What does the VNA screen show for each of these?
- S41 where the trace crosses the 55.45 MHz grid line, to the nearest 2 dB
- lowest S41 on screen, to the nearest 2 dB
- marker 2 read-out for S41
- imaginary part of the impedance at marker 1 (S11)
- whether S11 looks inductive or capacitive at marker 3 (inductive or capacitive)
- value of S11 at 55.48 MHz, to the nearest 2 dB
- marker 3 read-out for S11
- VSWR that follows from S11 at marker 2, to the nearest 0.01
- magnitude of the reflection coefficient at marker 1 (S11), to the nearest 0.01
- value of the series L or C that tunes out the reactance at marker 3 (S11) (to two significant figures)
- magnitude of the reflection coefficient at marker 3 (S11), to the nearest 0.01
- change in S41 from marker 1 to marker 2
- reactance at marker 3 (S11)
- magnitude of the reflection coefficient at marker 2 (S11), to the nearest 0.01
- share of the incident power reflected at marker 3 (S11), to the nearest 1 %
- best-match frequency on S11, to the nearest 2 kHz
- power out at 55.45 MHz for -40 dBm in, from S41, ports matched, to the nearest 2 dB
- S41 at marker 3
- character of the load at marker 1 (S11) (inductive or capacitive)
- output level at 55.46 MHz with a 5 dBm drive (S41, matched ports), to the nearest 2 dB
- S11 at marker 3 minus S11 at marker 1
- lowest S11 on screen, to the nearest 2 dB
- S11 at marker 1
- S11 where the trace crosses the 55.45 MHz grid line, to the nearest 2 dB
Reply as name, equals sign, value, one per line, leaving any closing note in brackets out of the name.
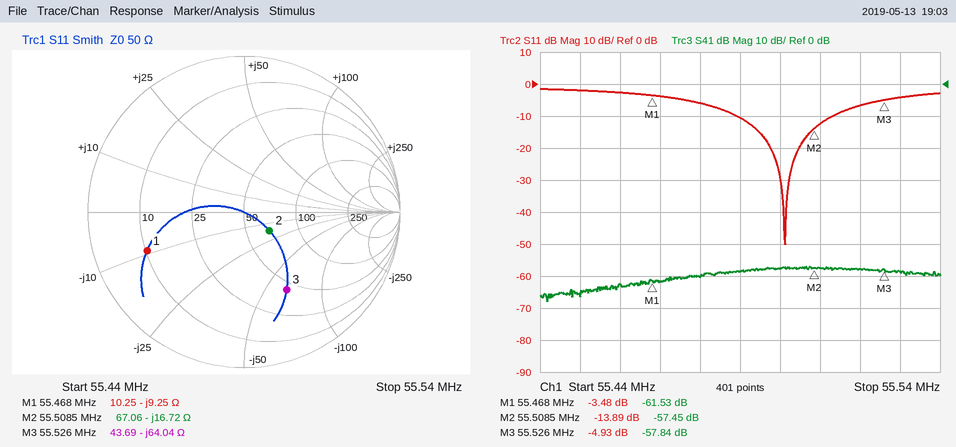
S41 where the trace crosses the 55.45 MHz grid line, to the nearest 2 dB = -66 dB
lowest S41 on screen, to the nearest 2 dB = -68 dB
marker 2 read-out for S41 = -57.45 dB
imaginary part of the impedance at marker 1 = -9.25 Ω
whether S11 looks inductive or capacitive at marker 3 = capacitive
value of S11 at 55.48 MHz, to the nearest 2 dB = -6 dB
marker 3 read-out for S11 = -4.93 dB
VSWR that follows from S11 at marker 2, to the nearest 0.01 = 1.51
magnitude of the reflection coefficient at marker 1 (S11), to the nearest 0.01 = 0.67
value of the series L or C that tunes out the reactance at marker 3 (S11) = 180 nH
magnitude of the reflection coefficient at marker 3 (S11), to the nearest 0.01 = 0.57
change in S41 from marker 1 to marker 2 = 4.08 dB
reactance at marker 3 = -64.04 Ω
magnitude of the reflection coefficient at marker 2 (S11), to the nearest 0.01 = 0.20
share of the incident power reflected at marker 3 (S11), to the nearest 1 % = 32 %
best-match frequency on S11, to the nearest 2 kHz = 55.502 MHz
power out at 55.45 MHz for -40 dBm in, from S41, ports matched, to the nearest 2 dB = -106 dBm
S41 at marker 3 = -57.84 dB
character of the load at marker 1 (S11) = capacitive
output level at 55.46 MHz with a 5 dBm drive (S41, matched ports), to the nearest 2 dB = -58 dBm
S11 at marker 3 minus S11 at marker 1 = -1.45 dB
lowest S11 on screen, to the nearest 2 dB = -50 dB
S11 at marker 1 = -3.48 dB
S11 where the trace crosses the 55.45 MHz grid line, to the nearest 2 dB = -2 dB
